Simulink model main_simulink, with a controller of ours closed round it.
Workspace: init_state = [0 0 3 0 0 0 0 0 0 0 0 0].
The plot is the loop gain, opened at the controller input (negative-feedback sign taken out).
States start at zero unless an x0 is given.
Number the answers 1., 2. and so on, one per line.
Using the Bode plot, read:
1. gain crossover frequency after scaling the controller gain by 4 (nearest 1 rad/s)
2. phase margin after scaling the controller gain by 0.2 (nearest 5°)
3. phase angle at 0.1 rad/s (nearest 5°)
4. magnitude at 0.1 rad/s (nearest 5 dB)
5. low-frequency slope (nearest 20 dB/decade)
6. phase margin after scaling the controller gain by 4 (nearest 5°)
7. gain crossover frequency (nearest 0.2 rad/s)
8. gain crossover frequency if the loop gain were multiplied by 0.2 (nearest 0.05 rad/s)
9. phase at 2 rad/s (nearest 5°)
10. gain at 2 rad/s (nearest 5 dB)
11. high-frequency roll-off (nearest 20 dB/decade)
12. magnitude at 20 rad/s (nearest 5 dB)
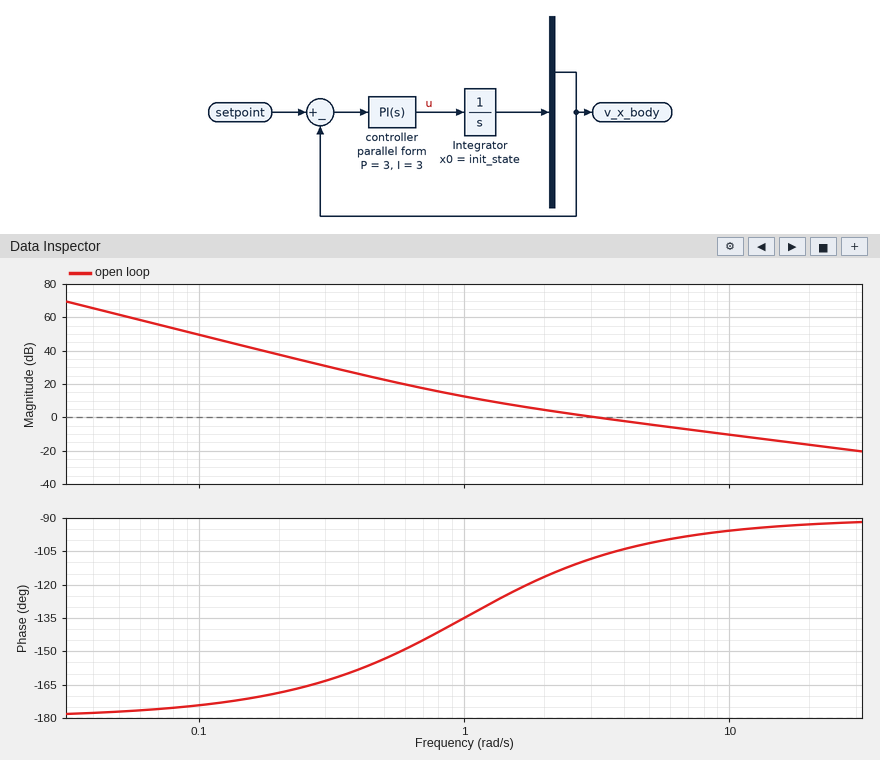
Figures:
1. 12 rad/s
2. 40°
3. -175°
4. 50 dB
5. -40 dB/decade
6. 85°
7. 3.2 rad/s
8. 0.90 rad/s
9. -115°
10. 5 dB
11. -20 dB/decade
12. -15 dB
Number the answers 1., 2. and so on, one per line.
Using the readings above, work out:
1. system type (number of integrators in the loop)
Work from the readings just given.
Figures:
1. 2
